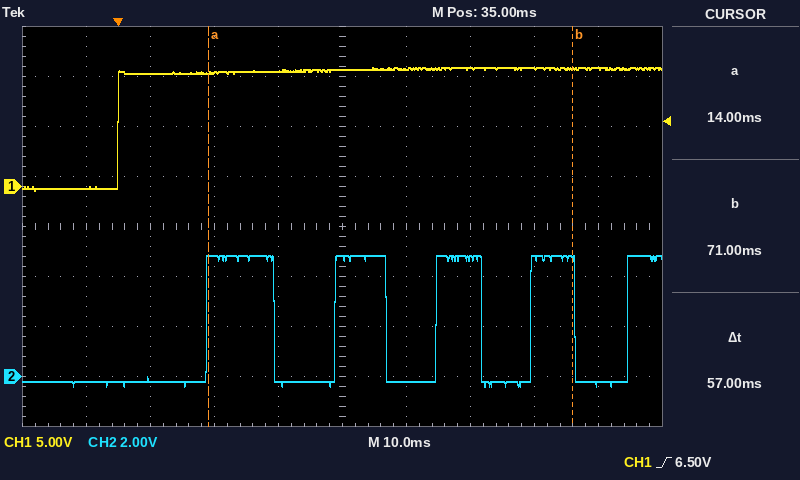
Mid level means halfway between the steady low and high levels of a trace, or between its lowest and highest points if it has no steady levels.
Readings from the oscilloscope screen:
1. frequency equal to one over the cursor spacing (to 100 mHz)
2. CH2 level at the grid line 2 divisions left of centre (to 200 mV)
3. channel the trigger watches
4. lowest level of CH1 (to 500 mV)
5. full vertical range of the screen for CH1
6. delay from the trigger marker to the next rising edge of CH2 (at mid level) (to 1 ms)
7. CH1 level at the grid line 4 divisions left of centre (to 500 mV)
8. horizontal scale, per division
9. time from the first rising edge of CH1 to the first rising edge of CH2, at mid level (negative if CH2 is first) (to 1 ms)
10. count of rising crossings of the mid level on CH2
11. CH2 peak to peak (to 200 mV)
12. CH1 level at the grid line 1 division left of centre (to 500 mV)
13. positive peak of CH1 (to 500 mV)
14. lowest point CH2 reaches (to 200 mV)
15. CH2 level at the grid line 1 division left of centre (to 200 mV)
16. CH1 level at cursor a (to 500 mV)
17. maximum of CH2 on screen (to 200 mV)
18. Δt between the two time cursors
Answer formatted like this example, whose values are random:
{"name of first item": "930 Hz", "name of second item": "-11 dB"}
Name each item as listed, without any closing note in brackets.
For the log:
{"frequency equal to one over the cursor spacing": "17.5 Hz", "CH2 level at the grid line 2 divisions left of centre": "4.8 V", "channel the trigger watches": "CH1", "lowest level of CH1": "-500 mV", "full vertical range of the screen for CH1": "40 V", "delay from the trigger marker to the next rising edge of CH2 (at mid level)": "14 ms", "CH1 level at the grid line 4 divisions left of centre": "0.0 V", "horizontal scale, per division": "10 ms", "time from the first rising edge of CH1 to the first rising edge of CH2, at mid level (negative if CH2 is first)": "+14 ms", "count of rising crossings of the mid level on CH2": "5", "CH2 peak to peak": "5.2 V", "CH1 level at the grid line 1 division left of centre": "11.5 V", "positive peak of CH1": "12.0 V", "lowest point CH2 reaches": "-400 mV", "CH2 level at the grid line 1 division left of centre": "-200 mV", "CH1 level at cursor a": "11.5 V", "maximum of CH2 on screen": "4.8 V", "Δt between the two time cursors": "57 ms"}
